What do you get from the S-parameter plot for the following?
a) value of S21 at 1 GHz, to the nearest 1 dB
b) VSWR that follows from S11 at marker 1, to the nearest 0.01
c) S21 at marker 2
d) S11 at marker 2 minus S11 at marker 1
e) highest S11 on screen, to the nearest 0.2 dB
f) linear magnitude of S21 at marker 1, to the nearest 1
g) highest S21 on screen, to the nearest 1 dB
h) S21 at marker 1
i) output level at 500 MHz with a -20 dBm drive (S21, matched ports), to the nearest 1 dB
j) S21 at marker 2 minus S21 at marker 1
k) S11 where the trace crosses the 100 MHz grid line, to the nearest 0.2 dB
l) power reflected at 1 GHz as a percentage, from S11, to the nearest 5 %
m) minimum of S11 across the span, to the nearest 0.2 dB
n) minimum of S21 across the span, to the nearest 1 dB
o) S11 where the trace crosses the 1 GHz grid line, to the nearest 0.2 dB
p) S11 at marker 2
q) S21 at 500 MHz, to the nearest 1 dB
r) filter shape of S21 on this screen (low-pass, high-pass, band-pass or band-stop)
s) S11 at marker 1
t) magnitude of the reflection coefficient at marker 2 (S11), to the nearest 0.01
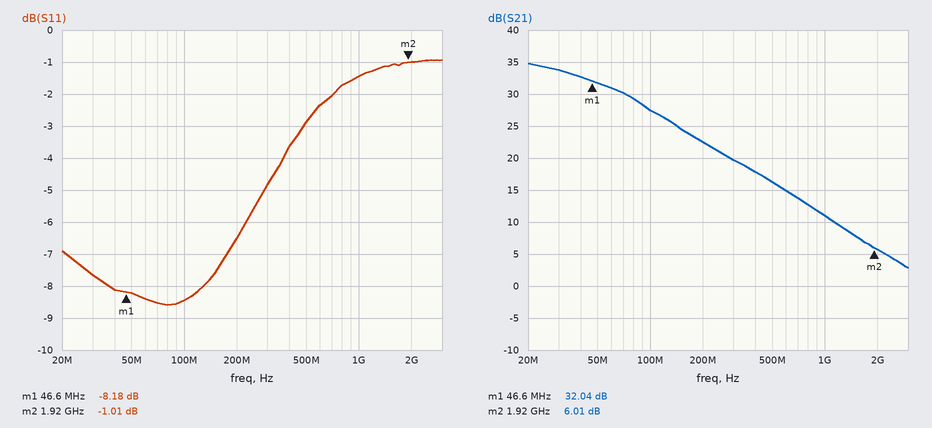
11 dB
2.28
6.01 dB
7.17 dB
-1.0 dB
40
35 dB
32.04 dB
-4 dBm
-26.03 dB
-8.4 dB
70 %
-8.6 dB
3 dB
-1.4 dB
-1.01 dB
16 dB
low-pass
-8.18 dB
0.89
